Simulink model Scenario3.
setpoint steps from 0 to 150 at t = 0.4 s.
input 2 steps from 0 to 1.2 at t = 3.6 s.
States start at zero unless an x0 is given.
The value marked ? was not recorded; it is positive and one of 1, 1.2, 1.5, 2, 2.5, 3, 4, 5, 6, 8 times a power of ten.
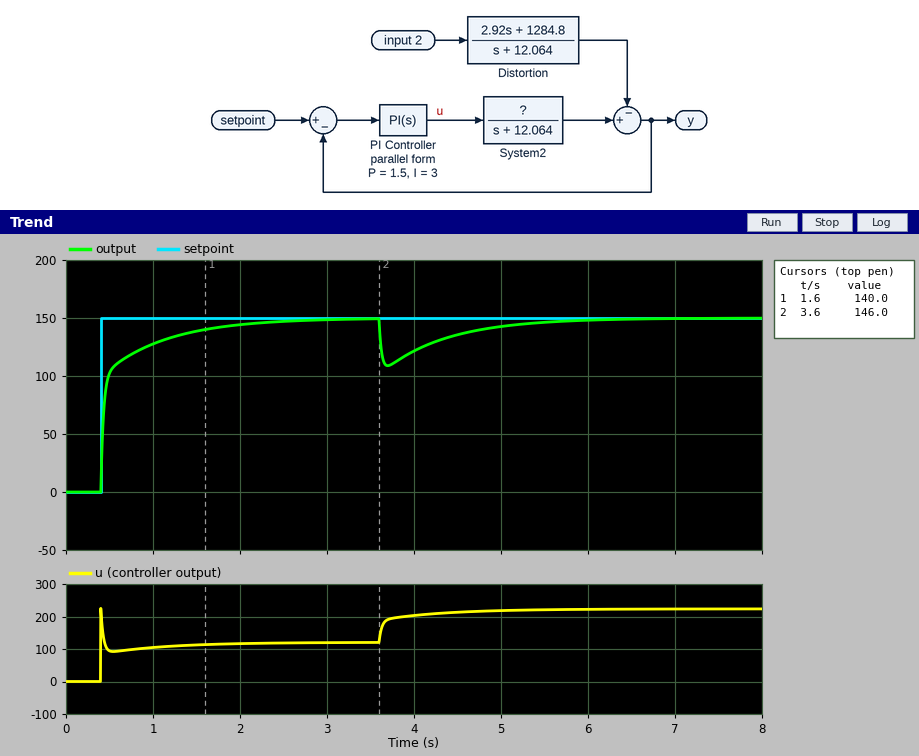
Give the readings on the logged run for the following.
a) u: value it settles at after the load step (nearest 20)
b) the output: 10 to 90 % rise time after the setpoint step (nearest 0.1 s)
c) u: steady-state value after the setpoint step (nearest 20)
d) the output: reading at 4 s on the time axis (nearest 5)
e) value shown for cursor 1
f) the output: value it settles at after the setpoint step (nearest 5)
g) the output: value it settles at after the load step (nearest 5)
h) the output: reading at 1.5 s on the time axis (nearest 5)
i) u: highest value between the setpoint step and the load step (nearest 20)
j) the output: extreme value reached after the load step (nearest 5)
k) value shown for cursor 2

220
0.9 s
120
120
140.0
150
150
140
220
110
146.0
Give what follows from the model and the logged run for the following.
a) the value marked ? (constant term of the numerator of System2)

15
